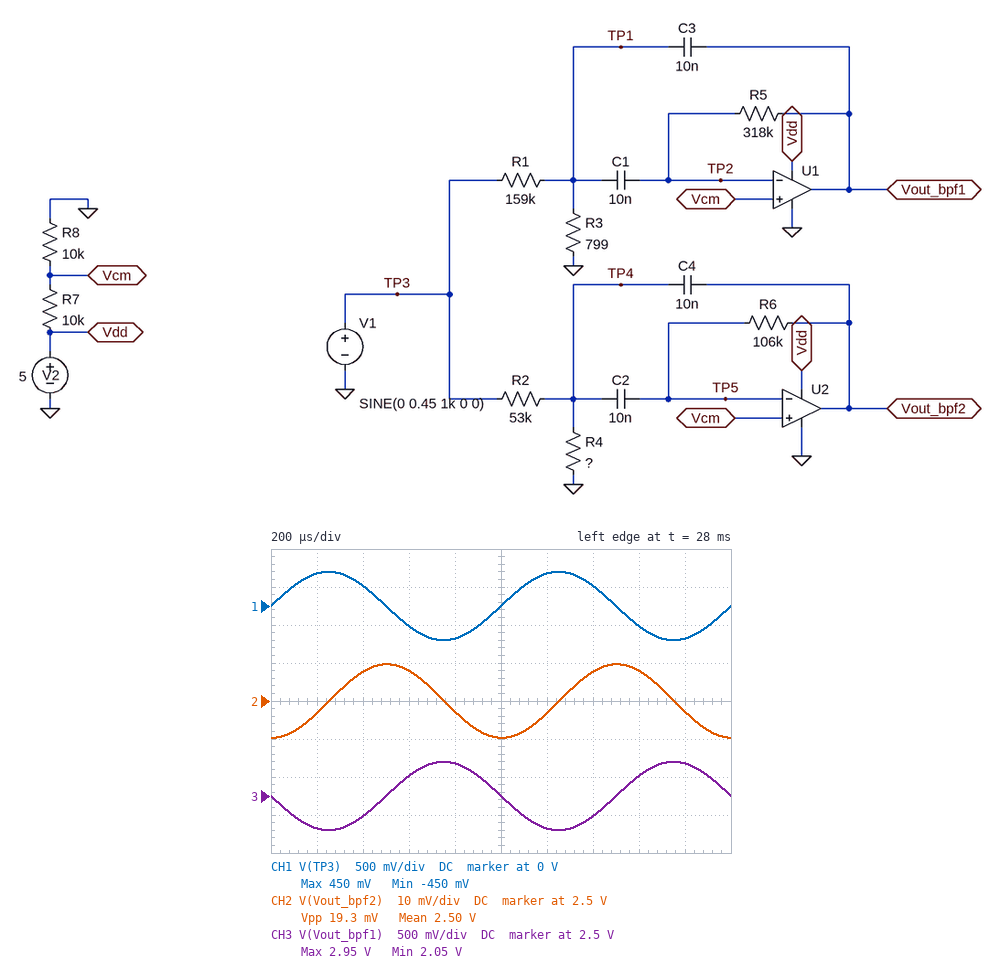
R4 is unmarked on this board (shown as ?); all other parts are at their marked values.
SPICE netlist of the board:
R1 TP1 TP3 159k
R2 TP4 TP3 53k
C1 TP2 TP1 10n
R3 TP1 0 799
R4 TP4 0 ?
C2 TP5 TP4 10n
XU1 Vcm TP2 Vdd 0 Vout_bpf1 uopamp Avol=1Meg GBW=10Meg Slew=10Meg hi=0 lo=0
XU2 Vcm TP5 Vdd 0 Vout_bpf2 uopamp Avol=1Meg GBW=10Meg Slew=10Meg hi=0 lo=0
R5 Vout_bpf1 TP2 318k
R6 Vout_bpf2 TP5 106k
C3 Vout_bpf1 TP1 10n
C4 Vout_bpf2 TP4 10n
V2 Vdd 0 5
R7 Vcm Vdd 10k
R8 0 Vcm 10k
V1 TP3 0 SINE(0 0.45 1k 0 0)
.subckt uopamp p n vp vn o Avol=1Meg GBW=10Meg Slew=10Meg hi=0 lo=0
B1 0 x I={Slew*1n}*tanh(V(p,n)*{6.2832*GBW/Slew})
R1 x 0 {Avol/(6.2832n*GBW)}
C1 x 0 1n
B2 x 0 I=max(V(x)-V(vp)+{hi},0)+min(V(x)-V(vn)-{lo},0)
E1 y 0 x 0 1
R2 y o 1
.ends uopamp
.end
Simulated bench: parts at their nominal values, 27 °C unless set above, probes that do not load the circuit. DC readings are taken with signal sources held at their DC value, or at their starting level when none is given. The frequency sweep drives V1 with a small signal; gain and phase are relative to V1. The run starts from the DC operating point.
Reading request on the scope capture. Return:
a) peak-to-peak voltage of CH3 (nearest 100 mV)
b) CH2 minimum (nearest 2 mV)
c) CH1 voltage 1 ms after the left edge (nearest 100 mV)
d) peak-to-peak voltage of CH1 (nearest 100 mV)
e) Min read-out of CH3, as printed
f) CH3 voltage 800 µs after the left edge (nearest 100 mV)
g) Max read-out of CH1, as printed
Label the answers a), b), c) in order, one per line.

a) 900 mV
b) 2.490 V
c) 0 V
d) 900 mV
e) 2.05 V
f) 2.9 V
g) 450 mV
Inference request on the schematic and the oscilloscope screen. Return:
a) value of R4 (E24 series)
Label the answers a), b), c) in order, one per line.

a) 160 Ω
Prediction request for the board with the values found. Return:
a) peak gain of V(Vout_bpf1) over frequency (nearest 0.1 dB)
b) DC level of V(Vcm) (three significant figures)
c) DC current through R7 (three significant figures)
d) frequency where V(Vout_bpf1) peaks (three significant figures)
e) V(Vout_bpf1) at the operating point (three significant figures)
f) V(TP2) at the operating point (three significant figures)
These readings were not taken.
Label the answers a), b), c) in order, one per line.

a) 0 dB
b) 2.50 V
c) 250 µA
d) 1.00 kHz
e) 2.50 V
f) 2.50 V
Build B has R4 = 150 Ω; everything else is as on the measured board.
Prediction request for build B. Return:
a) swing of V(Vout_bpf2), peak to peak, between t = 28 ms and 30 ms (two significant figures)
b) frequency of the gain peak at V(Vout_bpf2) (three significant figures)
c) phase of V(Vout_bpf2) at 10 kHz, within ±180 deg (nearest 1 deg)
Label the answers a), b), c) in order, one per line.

a) 18 mV
b) 3.98 kHz
c) 92 deg
